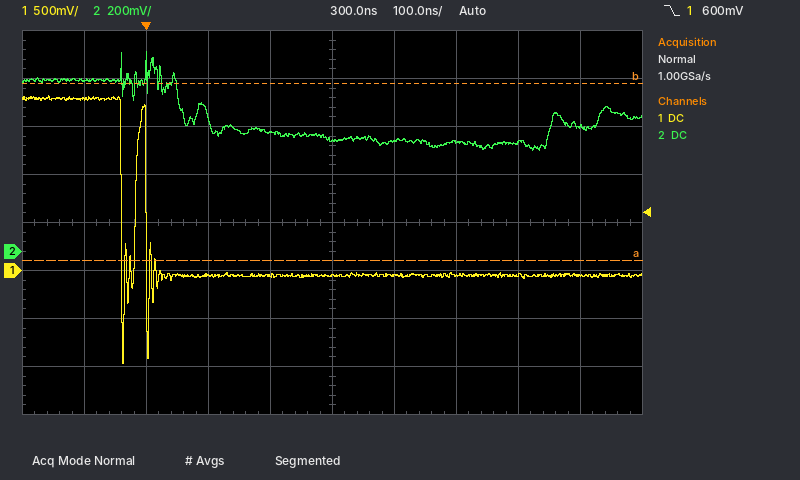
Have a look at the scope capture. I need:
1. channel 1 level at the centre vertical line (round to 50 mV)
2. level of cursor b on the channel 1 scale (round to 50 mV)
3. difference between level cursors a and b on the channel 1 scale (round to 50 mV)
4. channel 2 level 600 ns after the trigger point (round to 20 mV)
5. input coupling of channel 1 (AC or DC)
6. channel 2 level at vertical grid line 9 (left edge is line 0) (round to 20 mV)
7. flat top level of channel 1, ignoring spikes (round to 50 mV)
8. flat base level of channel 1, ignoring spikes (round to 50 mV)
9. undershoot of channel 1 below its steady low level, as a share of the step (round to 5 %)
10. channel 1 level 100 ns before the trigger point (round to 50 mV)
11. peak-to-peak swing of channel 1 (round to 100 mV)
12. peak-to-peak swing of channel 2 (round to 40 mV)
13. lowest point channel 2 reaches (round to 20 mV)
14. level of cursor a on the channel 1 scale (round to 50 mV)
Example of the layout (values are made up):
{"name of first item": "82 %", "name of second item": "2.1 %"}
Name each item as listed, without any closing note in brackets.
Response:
{"channel 1 level at the centre vertical line": "-50 mV", "level of cursor b on the channel 1 scale": "1.95 V", "difference between level cursors a and b on the channel 1 scale": "1.85 V", "channel 2 level 600 ns after the trigger point": "460 mV", "input coupling of channel 1": "DC", "channel 2 level at vertical grid line 9 (left edge is line 0)": "520 mV", "flat top level of channel 1, ignoring spikes": "1.80 V", "flat base level of channel 1, ignoring spikes": "-50 mV", "undershoot of channel 1 below its steady low level, as a share of the step": "50 %", "channel 1 level 100 ns before the trigger point": "1.80 V", "peak-to-peak swing of channel 1": "2.80 V", "peak-to-peak swing of channel 2": "400 mV", "lowest point channel 2 reaches": "420 mV", "level of cursor a on the channel 1 scale": "100 mV"}
